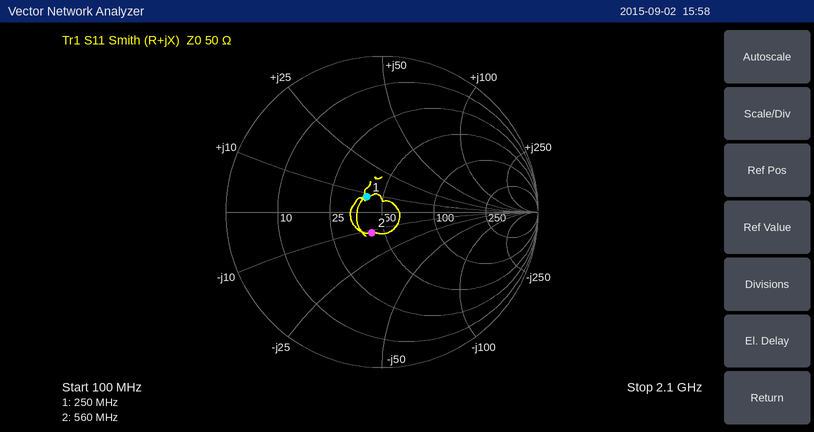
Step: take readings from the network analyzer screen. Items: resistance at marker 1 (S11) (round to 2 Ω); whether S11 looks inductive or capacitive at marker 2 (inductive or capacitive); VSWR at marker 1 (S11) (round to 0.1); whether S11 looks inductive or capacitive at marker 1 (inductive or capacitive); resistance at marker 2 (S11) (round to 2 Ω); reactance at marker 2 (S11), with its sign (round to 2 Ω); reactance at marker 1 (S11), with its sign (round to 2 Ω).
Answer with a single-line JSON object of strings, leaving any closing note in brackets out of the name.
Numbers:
{"resistance at marker 1 (S11)": "40 Ω", "whether S11 looks inductive or capacitive at marker 2": "capacitive", "VSWR at marker 1 (S11)": "1.3", "whether S11 looks inductive or capacitive at marker 1": "inductive", "resistance at marker 2 (S11)": "42 Ω", "reactance at marker 2 (S11), with its sign": "-12 Ω", "reactance at marker 1 (S11), with its sign": "+8 Ω"}
